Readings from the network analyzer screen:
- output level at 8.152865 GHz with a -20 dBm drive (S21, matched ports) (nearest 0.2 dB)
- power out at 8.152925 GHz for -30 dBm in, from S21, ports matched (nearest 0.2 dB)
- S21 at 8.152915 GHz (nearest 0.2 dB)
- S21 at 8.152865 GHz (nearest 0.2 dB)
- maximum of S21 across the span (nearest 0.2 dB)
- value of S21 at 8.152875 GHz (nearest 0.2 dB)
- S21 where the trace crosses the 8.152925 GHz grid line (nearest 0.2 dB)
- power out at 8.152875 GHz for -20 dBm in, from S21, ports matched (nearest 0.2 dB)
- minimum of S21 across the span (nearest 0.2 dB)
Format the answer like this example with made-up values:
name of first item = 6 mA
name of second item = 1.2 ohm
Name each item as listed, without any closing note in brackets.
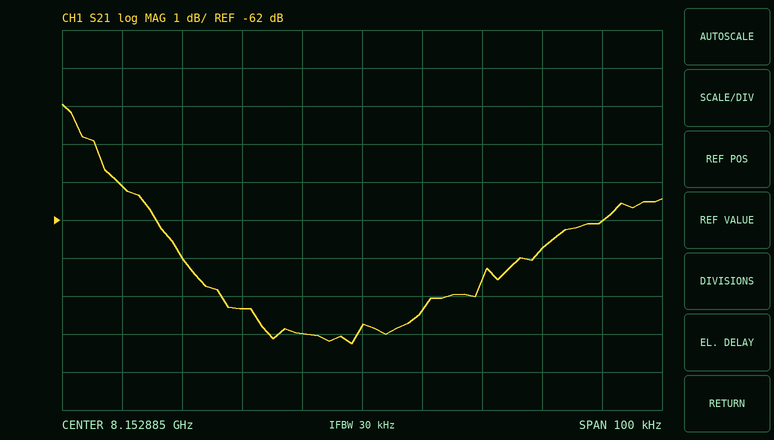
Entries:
output level at 8.152865 GHz with a -20 dBm drive (S21, matched ports) = -84.4 dBm
power out at 8.152925 GHz for -30 dBm in, from S21, ports matched = -92.0 dBm
S21 at 8.152915 GHz = -62.8 dB
S21 at 8.152865 GHz = -64.4 dB
maximum of S21 across the span = -59.0 dB
value of S21 at 8.152875 GHz = -65.0 dB
S21 where the trace crosses the 8.152925 GHz grid line = -62.0 dB
power out at 8.152875 GHz for -20 dBm in, from S21, ports matched = -85.0 dBm
minimum of S21 across the span = -65.2 dB
